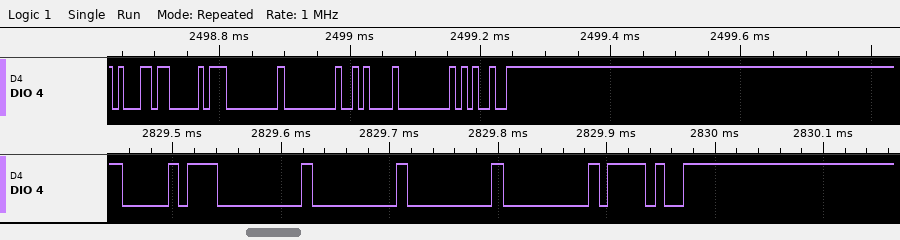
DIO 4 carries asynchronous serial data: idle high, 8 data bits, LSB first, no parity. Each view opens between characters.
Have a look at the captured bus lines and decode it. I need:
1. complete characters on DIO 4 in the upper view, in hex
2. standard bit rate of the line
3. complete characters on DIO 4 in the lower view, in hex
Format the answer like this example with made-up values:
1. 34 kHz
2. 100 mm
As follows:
1. B1, D0, 00, 00, 0A, 00, 25
2. 115200 baud
3. D0, 00, 00, 00, 00, 2F
